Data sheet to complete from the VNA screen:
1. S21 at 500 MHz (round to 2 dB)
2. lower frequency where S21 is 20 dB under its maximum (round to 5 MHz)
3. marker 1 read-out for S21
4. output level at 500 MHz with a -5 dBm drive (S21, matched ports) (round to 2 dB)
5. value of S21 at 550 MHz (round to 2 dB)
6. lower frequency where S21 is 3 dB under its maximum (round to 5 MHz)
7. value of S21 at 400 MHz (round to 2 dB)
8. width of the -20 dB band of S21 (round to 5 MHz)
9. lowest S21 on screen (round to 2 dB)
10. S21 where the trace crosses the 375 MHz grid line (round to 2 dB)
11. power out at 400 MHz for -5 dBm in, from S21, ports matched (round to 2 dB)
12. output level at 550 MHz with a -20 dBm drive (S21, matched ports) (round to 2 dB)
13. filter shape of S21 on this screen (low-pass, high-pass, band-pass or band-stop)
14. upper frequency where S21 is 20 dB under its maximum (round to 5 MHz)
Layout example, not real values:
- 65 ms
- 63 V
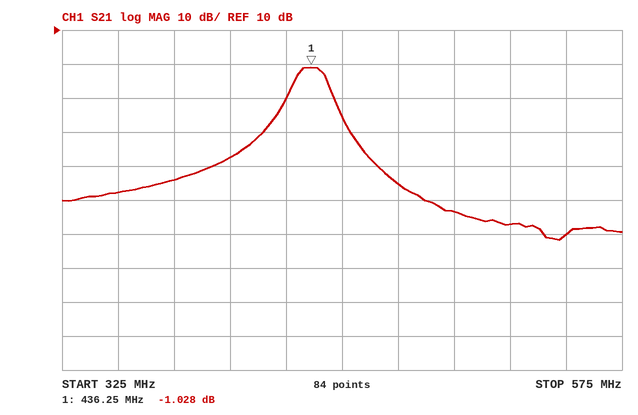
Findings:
- -44 dB
- 415 MHz
- -1.028 dB
- -48 dBm
- -50 dB
- 430 MHz
- -28 dB
- 40 MHz
- -52 dB
- -34 dB
- -32 dBm
- -70 dBm
- band-pass
- 455 MHz
